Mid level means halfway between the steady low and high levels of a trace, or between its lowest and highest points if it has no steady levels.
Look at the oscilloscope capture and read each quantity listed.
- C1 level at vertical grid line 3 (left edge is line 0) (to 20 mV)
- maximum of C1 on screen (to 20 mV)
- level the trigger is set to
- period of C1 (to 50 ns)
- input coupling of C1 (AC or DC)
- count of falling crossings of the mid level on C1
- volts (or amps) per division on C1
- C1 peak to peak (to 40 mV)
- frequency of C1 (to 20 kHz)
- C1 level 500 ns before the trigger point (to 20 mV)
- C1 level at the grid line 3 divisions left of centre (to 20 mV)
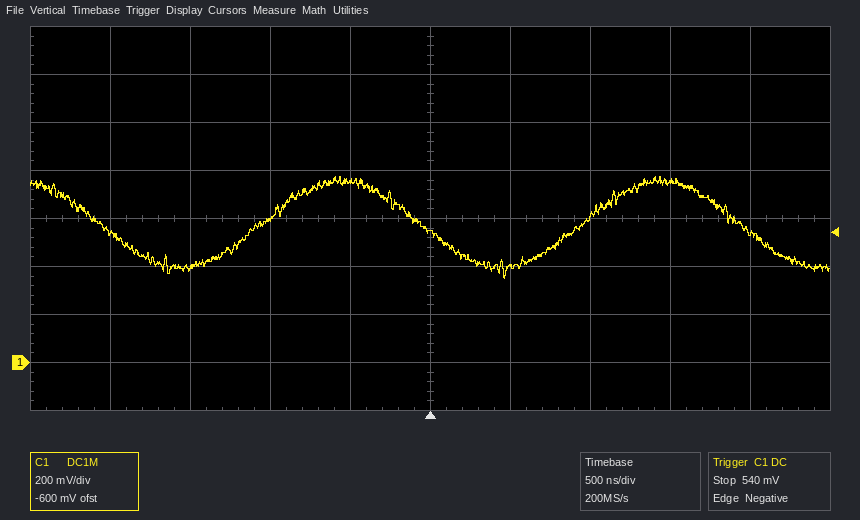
600 mV
780 mV
540 mV
2.00 µs
DC
3
200 mV
440 mV
500 kHz
760 mV
400 mV
